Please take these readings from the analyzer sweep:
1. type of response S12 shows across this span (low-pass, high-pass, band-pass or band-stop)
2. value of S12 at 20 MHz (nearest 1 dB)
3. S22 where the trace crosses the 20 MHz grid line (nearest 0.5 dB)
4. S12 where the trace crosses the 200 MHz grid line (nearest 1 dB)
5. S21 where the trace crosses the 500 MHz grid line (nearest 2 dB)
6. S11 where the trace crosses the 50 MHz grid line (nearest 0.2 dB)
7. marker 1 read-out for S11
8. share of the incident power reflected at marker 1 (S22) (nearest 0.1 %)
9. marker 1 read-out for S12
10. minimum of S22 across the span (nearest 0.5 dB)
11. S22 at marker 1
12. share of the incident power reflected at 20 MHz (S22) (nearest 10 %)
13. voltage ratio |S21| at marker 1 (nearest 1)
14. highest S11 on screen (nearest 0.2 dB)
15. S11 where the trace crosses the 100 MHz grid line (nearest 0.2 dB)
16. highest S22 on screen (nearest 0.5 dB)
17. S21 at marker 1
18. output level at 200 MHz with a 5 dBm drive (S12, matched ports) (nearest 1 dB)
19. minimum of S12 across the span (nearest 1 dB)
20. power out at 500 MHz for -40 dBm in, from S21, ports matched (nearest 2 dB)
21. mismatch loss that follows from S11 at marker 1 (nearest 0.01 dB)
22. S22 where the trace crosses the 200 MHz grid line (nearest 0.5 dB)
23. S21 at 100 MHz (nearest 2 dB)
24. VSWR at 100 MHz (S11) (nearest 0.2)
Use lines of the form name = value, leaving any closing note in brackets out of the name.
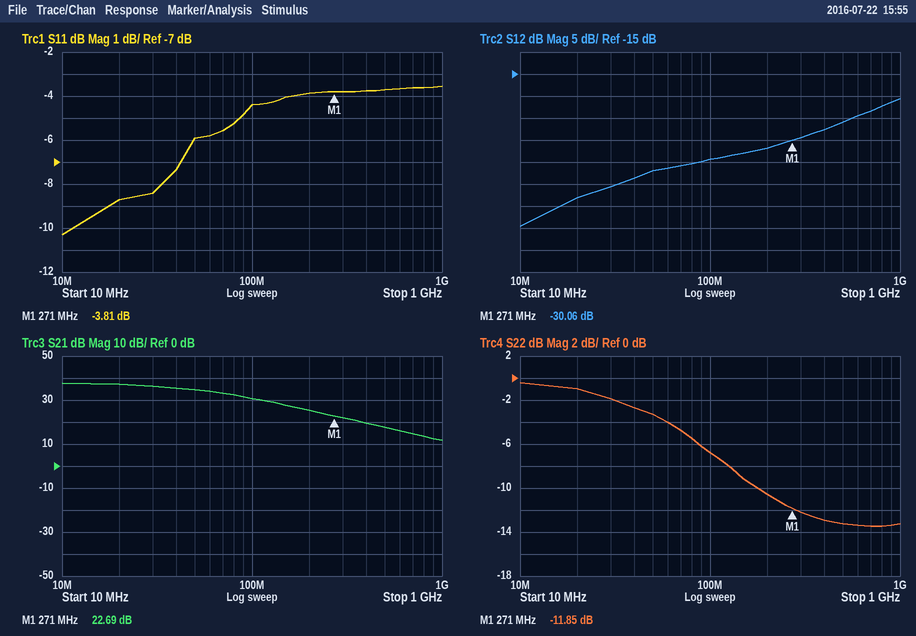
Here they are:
type of response S12 shows across this span = high-pass
value of S12 at 20 MHz = -43 dB
S22 where the trace crosses the 20 MHz grid line = -1.0 dB
S12 where the trace crosses the 200 MHz grid line = -32 dB
S21 where the trace crosses the 500 MHz grid line = 18 dB
S11 where the trace crosses the 50 MHz grid line = -6.0 dB
marker 1 read-out for S11 = -3.81 dB
share of the incident power reflected at marker 1 (S22) = 6.5 %
marker 1 read-out for S12 = -30.06 dB
minimum of S22 across the span = -13.5 dB
S22 at marker 1 = -11.85 dB
share of the incident power reflected at 20 MHz (S22) = 80 %
voltage ratio |S21| at marker 1 = 14
highest S11 on screen = -3.6 dB
S11 where the trace crosses the 100 MHz grid line = -4.4 dB
highest S22 on screen = -0.5 dB
S21 at marker 1 = 22.69 dB
output level at 200 MHz with a 5 dBm drive (S12, matched ports) = -27 dBm
minimum of S12 across the span = -50 dB
power out at 500 MHz for -40 dBm in, from S21, ports matched = -22 dBm
mismatch loss that follows from S11 at marker 1 = 2.34 dB
S22 where the trace crosses the 200 MHz grid line = -10.5 dB
S21 at 100 MHz = 30 dB
VSWR at 100 MHz (S11) = 4.0
